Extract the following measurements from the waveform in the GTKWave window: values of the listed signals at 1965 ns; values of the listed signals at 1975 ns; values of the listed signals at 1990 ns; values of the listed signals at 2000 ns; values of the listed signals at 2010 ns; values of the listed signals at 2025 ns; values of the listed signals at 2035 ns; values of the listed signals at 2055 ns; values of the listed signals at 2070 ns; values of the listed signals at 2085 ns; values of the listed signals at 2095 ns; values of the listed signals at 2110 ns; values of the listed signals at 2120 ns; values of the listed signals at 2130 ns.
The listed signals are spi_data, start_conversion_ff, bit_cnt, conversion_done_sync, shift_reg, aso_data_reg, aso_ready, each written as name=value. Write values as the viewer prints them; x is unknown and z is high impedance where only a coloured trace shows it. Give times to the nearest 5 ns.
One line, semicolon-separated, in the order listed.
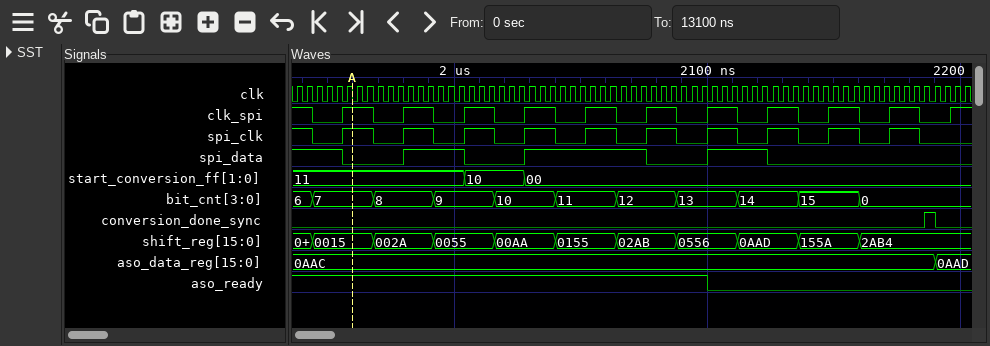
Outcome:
spi_data=0, start_conversion_ff=11, bit_cnt=7, conversion_done_sync=0, shift_reg=0015, aso_data_reg=0AAC, aso_ready=1; spi_data=0, start_conversion_ff=11, bit_cnt=8, conversion_done_sync=0, shift_reg=002A, aso_data_reg=0AAC, aso_ready=1; spi_data=1, start_conversion_ff=11, bit_cnt=8, conversion_done_sync=0, shift_reg=002A, aso_data_reg=0AAC, aso_ready=1; spi_data=1, start_conversion_ff=11, bit_cnt=9, conversion_done_sync=0, shift_reg=0055, aso_data_reg=0AAC, aso_ready=1; spi_data=0, start_conversion_ff=10, bit_cnt=9, conversion_done_sync=0, shift_reg=0055, aso_data_reg=0AAC, aso_ready=1; spi_data=0, start_conversion_ff=10, bit_cnt=10, conversion_done_sync=0, shift_reg=00AA, aso_data_reg=0AAC, aso_ready=1; spi_data=1, start_conversion_ff=00, bit_cnt=10, conversion_done_sync=0, shift_reg=00AA, aso_data_reg=0AAC, aso_ready=1; spi_data=1, start_conversion_ff=00, bit_cnt=11, conversion_done_sync=0, shift_reg=0155, aso_data_reg=0AAC, aso_ready=1; spi_data=1, start_conversion_ff=00, bit_cnt=12, conversion_done_sync=0, shift_reg=02AB, aso_data_reg=0AAC, aso_ready=1; spi_data=0, start_conversion_ff=00, bit_cnt=12, conversion_done_sync=0, shift_reg=02AB, aso_data_reg=0AAC, aso_ready=1; spi_data=0, start_conversion_ff=00, bit_cnt=13, conversion_done_sync=0, shift_reg=0556, aso_data_reg=0AAC, aso_ready=1; spi_data=1, start_conversion_ff=00, bit_cnt=13, conversion_done_sync=0, shift_reg=0556, aso_data_reg=0AAC, aso_ready=0; spi_data=1, start_conversion_ff=00, bit_cnt=14, conversion_done_sync=0, shift_reg=0AAD, aso_data_reg=0AAC, aso_ready=0; spi_data=0, start_conversion_ff=00, bit_cnt=14, conversion_done_sync=0, shift_reg=0AAD, aso_data_reg=0AAC, aso_ready=0
